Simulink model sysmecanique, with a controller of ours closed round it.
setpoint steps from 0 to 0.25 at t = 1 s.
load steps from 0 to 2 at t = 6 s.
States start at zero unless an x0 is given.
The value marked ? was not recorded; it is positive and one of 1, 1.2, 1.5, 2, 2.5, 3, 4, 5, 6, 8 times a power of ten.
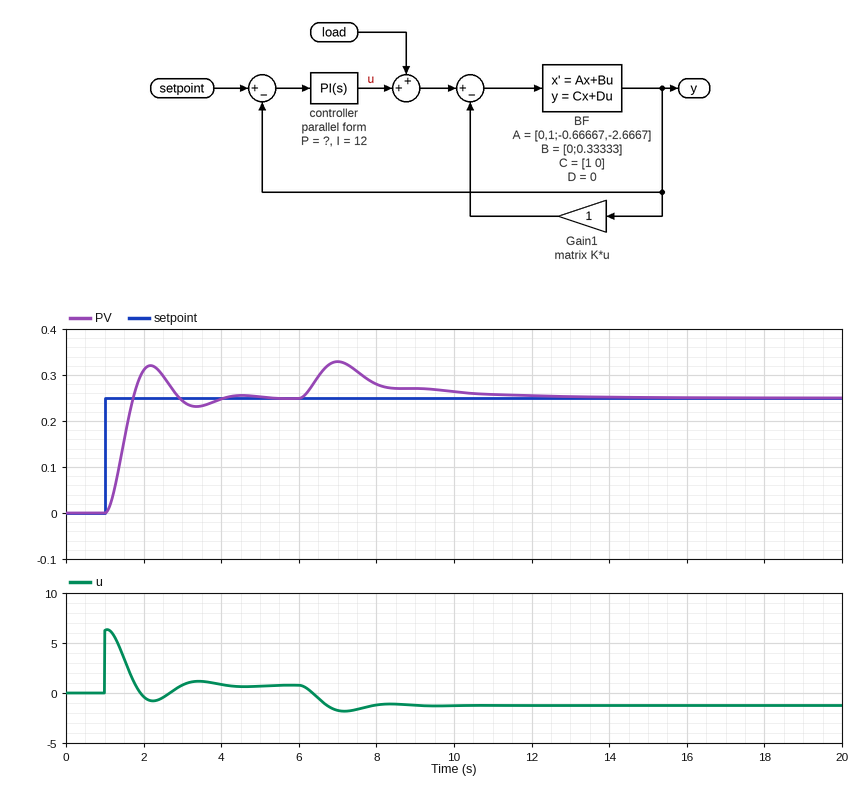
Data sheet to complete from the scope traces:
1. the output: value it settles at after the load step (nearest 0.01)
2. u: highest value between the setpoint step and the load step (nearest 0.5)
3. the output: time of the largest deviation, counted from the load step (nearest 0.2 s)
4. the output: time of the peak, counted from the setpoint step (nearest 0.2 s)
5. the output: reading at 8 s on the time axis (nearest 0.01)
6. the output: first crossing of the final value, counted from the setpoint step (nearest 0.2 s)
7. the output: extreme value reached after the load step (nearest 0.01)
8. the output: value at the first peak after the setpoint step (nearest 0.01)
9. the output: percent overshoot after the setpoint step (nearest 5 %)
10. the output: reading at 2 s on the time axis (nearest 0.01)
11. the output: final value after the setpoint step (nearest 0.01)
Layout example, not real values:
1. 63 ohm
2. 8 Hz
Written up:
1. 0.25
2. 6.5
3. 1.0 s
4. 1.2 s
5. 0.28
6. 0.8 s
7. 0.33
8. 0.32
9. 30 %
10. 0.31
11. 0.25
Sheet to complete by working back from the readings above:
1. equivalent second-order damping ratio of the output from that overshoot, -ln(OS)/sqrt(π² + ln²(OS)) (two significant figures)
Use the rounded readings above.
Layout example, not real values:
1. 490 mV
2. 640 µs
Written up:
1. 0.36
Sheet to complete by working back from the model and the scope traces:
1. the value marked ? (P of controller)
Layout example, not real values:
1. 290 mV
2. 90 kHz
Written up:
1. 25
